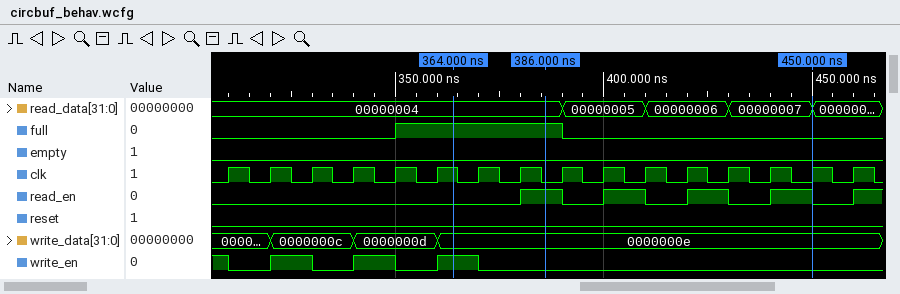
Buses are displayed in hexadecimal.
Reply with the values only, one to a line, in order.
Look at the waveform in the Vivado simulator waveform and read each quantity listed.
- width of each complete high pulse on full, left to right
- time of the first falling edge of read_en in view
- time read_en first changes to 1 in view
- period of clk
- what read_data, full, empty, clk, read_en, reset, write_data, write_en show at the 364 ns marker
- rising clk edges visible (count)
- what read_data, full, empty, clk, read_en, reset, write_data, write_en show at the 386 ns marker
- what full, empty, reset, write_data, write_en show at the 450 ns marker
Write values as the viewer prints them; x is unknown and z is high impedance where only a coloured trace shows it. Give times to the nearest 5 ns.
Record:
40 ns
390 ns
380 ns
10 ns
read_data=00000004, full=1, empty=0, clk=1, read_en=0, reset=0, write_data=0000000e, write_en=1
16
read_data=00000004, full=1, empty=0, clk=0, read_en=1, reset=0, write_data=0000000e, write_en=0
full=0, empty=0, reset=0, write_data=0000000e, write_en=0
